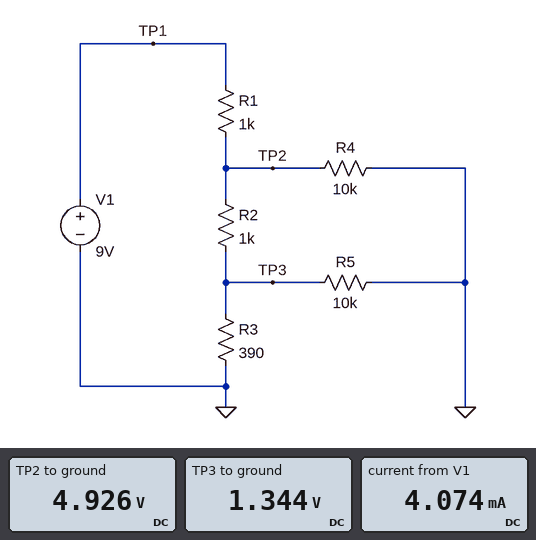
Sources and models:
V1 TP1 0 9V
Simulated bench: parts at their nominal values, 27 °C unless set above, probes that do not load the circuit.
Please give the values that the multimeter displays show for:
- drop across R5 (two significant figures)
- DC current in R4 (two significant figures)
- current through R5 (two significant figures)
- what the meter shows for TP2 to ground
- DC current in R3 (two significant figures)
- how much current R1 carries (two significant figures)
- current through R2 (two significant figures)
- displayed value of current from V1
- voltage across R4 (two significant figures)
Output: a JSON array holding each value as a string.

["1.3 V", "490 µA", "130 µA", "4.926 V", "3.4 mA", "4.1 mA", "3.6 mA", "4.074 mA", "4.9 V"]
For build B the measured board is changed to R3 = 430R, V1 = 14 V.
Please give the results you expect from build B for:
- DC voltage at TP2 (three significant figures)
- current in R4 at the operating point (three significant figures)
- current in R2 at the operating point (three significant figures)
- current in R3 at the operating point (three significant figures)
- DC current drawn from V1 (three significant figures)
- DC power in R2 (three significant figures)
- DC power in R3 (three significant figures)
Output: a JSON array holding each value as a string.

["7.74 V", "774 µA", "5.48 mA", "5.26 mA", "6.26 mA", "30.1 mW", "11.9 mW"]
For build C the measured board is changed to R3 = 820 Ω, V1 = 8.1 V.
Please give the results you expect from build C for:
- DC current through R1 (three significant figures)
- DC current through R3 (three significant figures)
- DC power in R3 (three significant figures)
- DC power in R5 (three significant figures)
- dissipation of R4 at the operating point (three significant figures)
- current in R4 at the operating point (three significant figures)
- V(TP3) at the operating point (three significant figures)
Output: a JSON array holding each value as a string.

["3.25 mA", "2.55 mA", "5.34 mW", "438 µW", "2.36 mW", "485 µA", "2.09 V"]
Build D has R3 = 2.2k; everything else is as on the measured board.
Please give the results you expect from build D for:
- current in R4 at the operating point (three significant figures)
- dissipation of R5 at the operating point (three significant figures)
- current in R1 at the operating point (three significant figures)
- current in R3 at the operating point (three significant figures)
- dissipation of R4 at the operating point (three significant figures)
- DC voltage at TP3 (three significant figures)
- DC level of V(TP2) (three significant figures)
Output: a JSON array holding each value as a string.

["618 µA", "1.58 mW", "2.82 mA", "1.81 mA", "3.82 mW", "3.97 V", "6.18 V"]
